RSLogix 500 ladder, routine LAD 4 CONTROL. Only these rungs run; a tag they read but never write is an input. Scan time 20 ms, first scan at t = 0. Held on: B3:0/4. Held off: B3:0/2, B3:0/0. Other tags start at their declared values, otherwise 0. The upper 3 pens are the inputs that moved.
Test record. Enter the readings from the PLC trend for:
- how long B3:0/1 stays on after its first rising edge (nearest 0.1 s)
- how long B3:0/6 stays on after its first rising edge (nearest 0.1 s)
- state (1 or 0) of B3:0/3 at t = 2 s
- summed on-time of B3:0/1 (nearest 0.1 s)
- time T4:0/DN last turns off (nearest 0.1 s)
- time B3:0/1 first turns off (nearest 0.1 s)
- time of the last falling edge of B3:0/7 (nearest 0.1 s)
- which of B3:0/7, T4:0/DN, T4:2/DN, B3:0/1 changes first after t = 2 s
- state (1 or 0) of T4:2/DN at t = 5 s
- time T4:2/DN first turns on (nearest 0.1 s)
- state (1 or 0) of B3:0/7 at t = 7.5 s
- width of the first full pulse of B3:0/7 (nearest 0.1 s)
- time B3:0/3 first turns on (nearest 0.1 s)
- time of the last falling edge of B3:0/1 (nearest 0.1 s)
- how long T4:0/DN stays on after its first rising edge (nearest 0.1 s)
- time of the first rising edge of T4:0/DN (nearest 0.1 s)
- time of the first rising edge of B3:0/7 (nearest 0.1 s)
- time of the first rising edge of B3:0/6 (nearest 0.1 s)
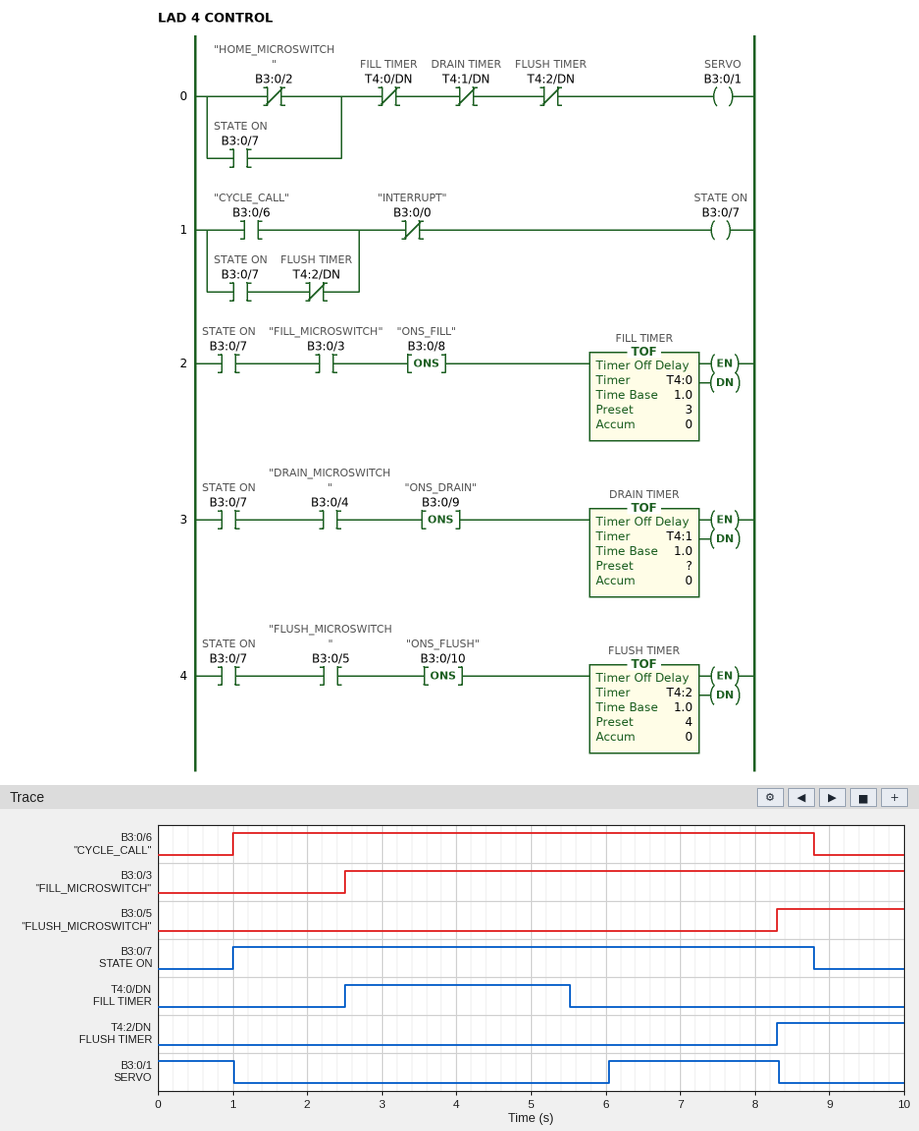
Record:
2.3 s
7.8 s
0
3.3 s
5.5 s
1.0 s
8.8 s
T4:0/DN
0
8.3 s
1
7.8 s
2.5 s
8.3 s
3.0 s
2.5 s
1.0 s
1.0 s
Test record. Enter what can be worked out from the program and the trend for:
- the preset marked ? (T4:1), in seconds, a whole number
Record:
5 s
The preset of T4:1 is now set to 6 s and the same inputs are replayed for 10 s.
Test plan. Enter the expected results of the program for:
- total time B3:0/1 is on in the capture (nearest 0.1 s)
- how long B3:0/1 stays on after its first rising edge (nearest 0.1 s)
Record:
2.3 s
1.3 s
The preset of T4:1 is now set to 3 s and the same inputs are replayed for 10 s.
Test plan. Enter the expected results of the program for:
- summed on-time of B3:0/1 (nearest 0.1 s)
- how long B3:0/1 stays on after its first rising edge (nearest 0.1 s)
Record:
3.8 s
2.8 s
